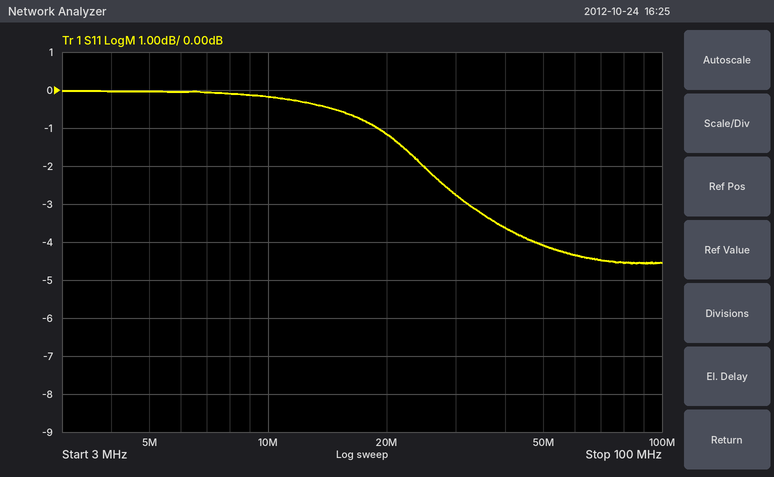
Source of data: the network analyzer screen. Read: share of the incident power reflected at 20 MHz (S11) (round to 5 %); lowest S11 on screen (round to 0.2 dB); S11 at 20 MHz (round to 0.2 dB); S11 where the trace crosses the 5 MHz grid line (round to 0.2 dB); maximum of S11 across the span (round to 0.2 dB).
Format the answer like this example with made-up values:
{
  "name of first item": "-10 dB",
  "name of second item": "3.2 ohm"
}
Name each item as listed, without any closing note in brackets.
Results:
{
  "share of the incident power reflected at 20 MHz (S11)": "75 %",
  "lowest S11 on screen": "-4.6 dB",
  "S11 at 20 MHz": "-1.2 dB",
  "S11 where the trace crosses the 5 MHz grid line": "0.0 dB",
  "maximum of S11 across the span": "0.0 dB"
}
